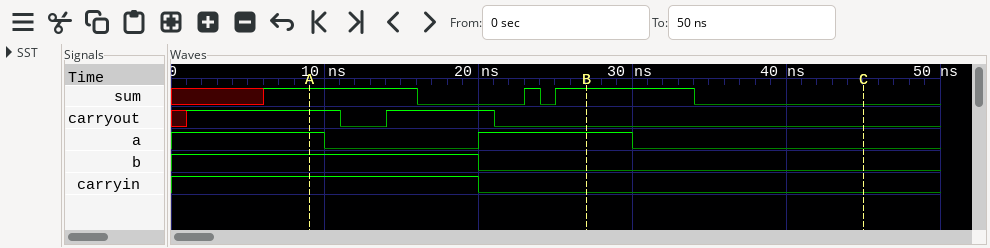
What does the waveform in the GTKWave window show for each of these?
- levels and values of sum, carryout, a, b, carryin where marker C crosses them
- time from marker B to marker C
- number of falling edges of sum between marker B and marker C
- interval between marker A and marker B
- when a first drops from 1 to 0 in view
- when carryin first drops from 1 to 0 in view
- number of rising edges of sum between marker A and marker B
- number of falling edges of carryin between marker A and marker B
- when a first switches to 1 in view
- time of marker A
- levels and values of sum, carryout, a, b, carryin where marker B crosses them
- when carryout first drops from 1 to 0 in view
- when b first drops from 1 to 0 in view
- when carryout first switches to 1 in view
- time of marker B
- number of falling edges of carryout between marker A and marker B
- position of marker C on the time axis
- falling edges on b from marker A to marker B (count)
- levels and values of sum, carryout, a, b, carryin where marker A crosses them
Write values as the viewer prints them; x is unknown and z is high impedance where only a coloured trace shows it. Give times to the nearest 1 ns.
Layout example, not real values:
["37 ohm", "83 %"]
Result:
["sum=0, carryout=0, a=0, b=0, carryin=0", "18 ns", "1", "18 ns", "10 ns", "20 ns", "2", "1", "20 ns", "9 ns", "sum=1, carryout=0, a=1, b=0, carryin=0", "11 ns", "20 ns", "1 ns", "27 ns", "2", "45 ns", "1", "sum=1, carryout=1, a=1, b=1, carryin=1"]
